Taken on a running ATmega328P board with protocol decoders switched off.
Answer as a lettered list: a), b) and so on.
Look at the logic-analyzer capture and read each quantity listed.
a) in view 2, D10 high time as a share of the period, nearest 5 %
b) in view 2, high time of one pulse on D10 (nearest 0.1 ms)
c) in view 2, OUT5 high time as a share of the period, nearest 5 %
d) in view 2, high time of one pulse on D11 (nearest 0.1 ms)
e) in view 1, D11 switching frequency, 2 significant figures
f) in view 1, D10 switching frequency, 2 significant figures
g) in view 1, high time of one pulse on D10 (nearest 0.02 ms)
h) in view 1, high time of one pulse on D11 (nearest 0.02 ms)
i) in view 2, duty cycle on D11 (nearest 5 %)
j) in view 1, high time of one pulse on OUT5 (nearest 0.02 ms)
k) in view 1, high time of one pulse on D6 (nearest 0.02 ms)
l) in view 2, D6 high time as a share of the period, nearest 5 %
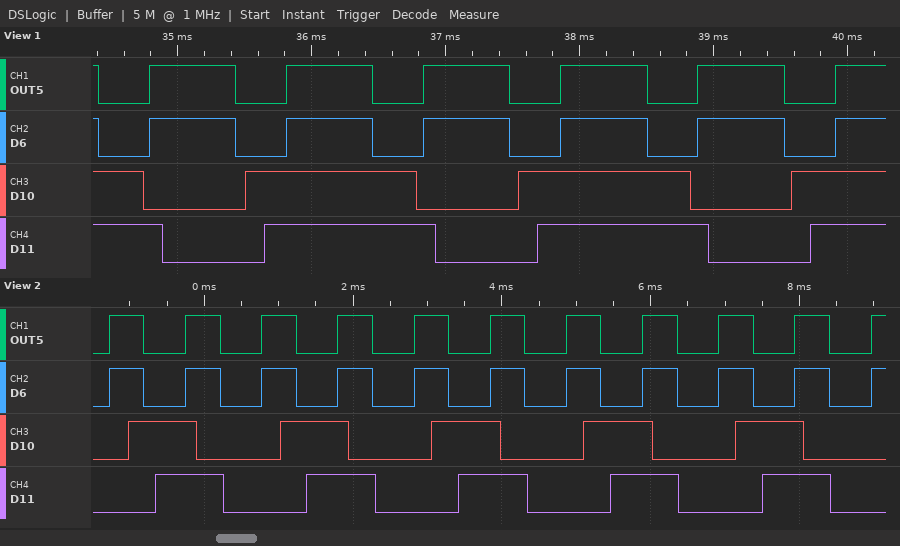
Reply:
a) 45 %
b) 0.9 ms
c) 45 %
d) 0.9 ms
e) 490 Hz
f) 490 Hz
g) 1.28 ms
h) 1.28 ms
i) 45 %
j) 0.64 ms
k) 0.64 ms
l) 45 %
